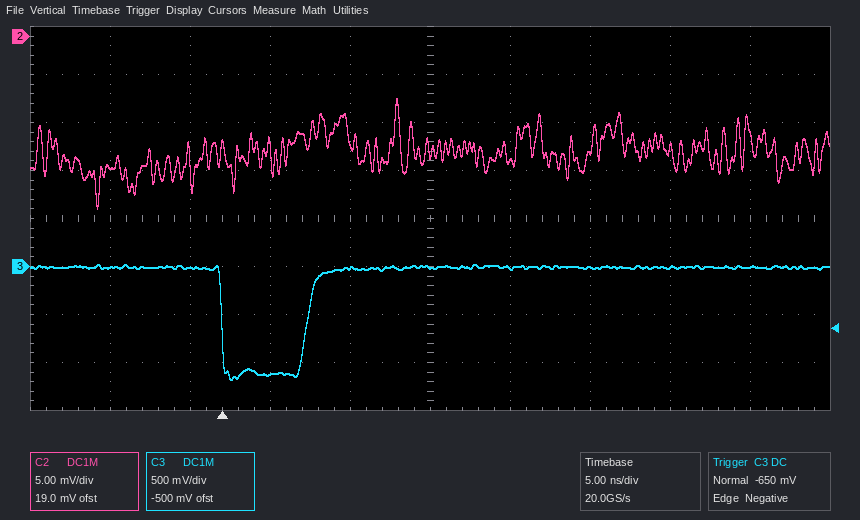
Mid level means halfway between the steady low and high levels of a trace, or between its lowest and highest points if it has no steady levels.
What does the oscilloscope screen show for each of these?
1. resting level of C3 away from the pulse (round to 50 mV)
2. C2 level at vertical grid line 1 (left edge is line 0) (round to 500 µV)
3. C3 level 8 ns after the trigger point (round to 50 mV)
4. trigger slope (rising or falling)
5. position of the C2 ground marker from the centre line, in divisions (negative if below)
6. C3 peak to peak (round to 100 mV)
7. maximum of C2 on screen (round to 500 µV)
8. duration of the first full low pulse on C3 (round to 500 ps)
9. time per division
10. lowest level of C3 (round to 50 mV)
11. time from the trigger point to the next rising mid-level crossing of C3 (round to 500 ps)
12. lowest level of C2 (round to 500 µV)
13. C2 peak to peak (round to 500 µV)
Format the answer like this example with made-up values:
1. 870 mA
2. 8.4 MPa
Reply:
1. 0 mV
2. -13.5 mV
3. 0 mV
4. falling
5. +3.8 div
6. 1.20 V
7. -6.5 mV
8. 5.5 ns
9. 5 ns
10. -1.20 V
11. 5.5 ns
12. -18.0 mV
13. 11.5 mV
